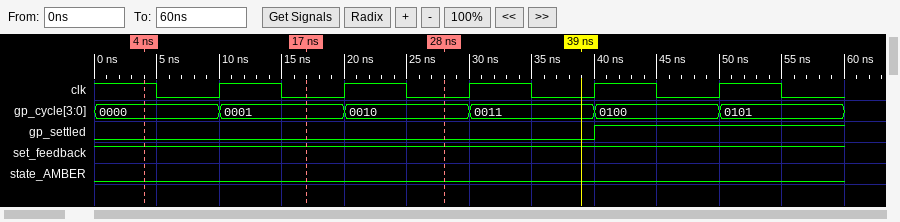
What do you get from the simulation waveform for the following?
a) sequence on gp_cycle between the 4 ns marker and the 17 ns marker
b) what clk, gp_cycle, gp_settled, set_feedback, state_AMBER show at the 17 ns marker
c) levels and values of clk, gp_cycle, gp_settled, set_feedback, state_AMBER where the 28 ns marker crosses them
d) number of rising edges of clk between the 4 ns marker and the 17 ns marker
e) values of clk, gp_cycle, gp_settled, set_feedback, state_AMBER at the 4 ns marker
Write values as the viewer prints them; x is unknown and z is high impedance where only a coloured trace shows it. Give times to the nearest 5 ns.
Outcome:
0000, 0001
clk=0, gp_cycle=0001, gp_settled=0, set_feedback=1, state_AMBER=0
clk=0, gp_cycle=0010, gp_settled=0, set_feedback=1, state_AMBER=0
1
clk=1, gp_cycle=0000, gp_settled=0, set_feedback=1, state_AMBER=0
